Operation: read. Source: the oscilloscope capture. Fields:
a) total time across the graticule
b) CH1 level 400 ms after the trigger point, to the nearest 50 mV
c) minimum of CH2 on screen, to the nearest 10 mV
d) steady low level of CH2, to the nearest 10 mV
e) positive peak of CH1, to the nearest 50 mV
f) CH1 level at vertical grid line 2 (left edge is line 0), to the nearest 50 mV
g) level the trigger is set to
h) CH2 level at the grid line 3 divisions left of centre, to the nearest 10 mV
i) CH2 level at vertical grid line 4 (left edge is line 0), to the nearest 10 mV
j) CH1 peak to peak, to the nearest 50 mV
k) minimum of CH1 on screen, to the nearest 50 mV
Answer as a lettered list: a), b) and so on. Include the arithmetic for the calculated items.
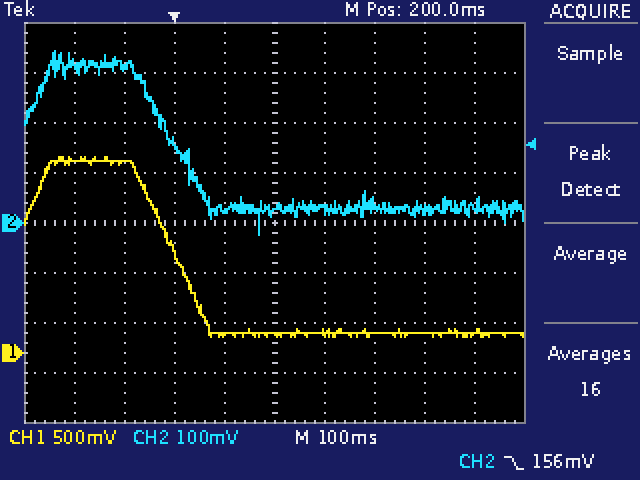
a) 1 s
b) 200 mV
c) -20 mV
d) 30 mV
e) 1.95 V
f) 1.90 V
g) 156 mV
h) 310 mV
i) 30 mV
j) 1.95 V − (150 mV) = 1.80 V
k) 150 mV
